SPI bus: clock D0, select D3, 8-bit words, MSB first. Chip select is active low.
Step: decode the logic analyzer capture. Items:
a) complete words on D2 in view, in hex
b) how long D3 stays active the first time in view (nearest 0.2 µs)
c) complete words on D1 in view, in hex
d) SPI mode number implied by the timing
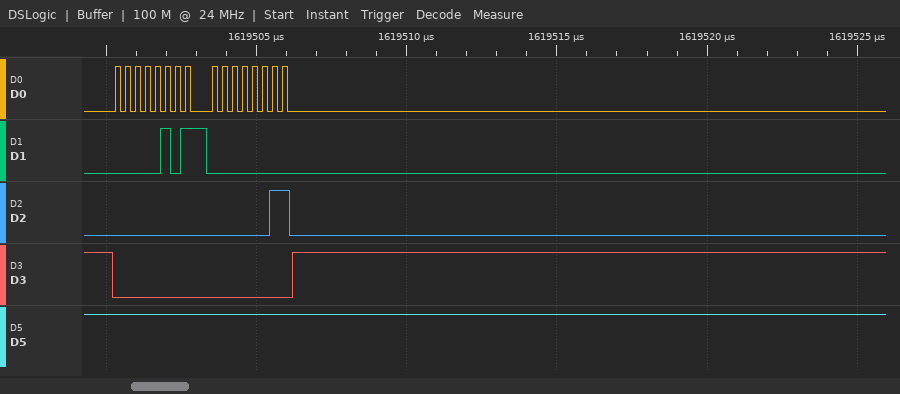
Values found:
00, 03
6 µs
05, 00
0
